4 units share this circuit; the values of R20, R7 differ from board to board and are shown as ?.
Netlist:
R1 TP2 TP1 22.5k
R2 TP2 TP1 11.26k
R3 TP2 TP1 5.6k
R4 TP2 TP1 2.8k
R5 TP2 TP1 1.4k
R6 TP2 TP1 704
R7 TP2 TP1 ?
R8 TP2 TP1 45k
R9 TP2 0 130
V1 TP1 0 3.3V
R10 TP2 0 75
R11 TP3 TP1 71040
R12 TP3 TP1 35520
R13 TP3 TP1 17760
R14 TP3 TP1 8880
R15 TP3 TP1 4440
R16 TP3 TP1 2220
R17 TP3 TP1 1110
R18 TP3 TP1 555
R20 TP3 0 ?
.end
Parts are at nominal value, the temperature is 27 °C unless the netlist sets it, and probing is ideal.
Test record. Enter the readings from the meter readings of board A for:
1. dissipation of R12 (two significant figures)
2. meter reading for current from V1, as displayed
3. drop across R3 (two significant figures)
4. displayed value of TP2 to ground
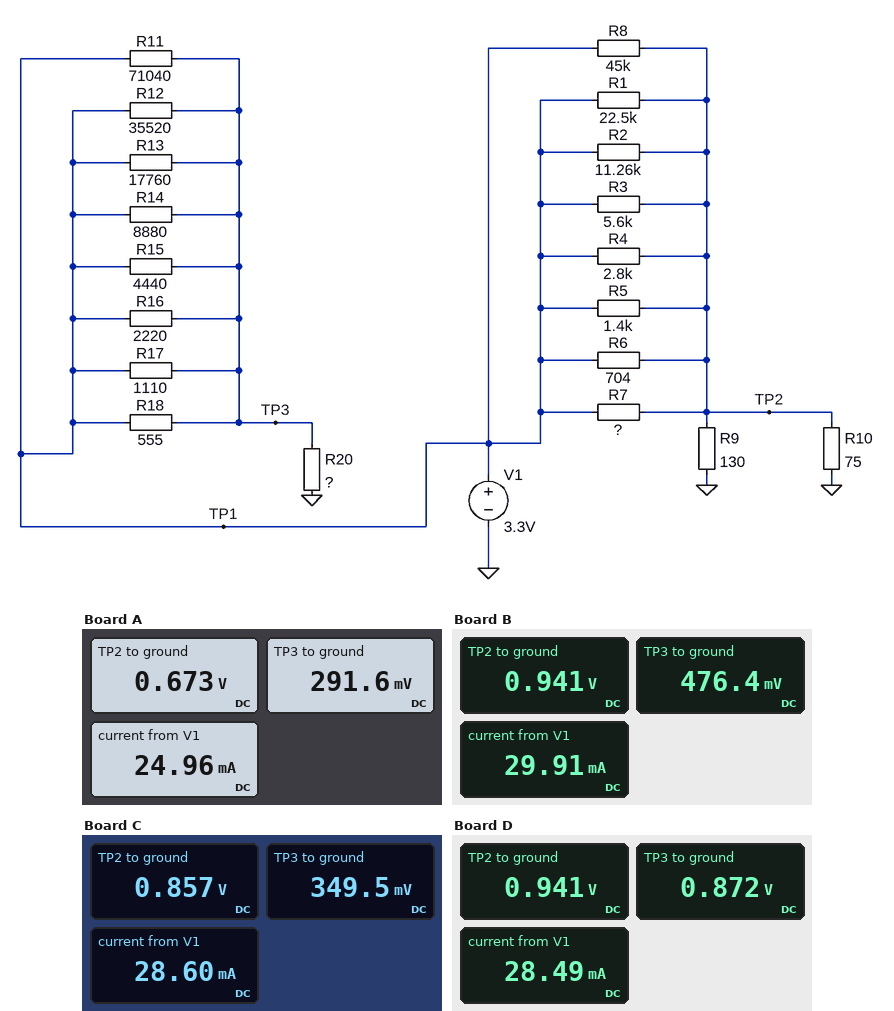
250 µW
24.96 mA
2.6 V
0.673 V
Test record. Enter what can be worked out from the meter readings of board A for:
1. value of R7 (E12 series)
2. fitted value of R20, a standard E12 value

390 Ω
27 Ω
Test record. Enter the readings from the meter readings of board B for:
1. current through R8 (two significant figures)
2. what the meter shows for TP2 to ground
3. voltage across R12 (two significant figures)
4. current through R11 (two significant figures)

52 µA
0.941 V
2.8 V
40 µA
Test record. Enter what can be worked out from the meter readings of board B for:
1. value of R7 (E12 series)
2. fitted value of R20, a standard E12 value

180 Ω
47 Ω
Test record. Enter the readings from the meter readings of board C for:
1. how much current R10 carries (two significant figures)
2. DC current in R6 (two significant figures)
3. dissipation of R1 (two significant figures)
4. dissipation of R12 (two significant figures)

11 mA
3.5 mA
270 µW
250 µW
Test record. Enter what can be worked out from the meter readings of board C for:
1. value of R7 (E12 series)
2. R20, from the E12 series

220 Ω
33 Ω
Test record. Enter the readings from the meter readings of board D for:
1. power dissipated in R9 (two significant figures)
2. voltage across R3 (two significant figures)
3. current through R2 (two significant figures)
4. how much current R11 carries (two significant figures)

6.8 mW
2.4 V
210 µA
34 µA
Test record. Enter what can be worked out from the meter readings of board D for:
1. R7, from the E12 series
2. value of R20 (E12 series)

180 Ω
100 Ω
